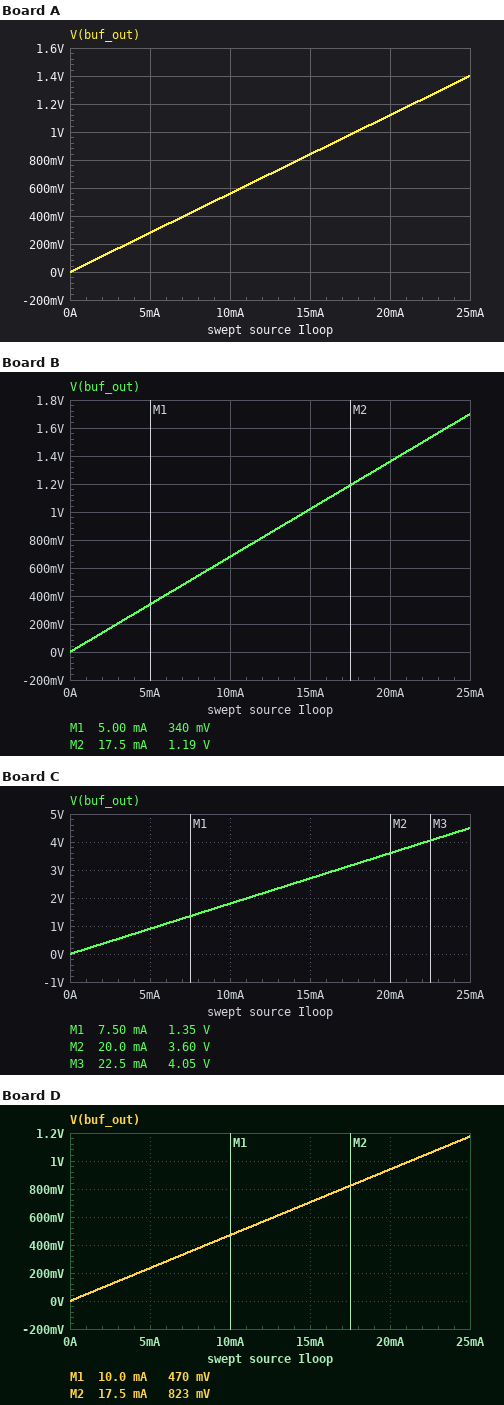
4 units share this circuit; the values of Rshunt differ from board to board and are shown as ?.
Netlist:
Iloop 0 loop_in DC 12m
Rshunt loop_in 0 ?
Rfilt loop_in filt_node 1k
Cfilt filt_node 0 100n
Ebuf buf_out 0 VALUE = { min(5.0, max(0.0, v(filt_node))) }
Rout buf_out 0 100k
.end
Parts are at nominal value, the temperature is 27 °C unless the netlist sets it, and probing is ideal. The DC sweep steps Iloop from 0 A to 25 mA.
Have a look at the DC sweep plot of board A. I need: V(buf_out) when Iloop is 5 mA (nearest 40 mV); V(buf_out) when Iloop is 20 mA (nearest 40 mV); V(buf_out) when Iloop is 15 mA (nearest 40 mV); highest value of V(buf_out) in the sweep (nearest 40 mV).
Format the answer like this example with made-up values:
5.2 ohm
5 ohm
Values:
280 mV
1.12 V
840 mV
1.40 V
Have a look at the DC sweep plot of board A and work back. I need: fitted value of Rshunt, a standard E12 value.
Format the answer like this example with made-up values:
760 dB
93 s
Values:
56 Ω
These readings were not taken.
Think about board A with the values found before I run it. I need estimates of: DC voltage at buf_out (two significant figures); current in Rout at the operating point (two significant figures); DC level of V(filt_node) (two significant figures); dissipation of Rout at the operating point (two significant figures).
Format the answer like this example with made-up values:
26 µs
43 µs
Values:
670 mV
6.7 µA
670 mV
4.5 µW
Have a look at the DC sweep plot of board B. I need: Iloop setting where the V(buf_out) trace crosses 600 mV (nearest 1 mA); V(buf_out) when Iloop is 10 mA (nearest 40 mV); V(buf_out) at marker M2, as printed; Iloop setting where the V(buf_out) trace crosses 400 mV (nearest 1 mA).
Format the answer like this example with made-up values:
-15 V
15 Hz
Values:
9 mA
680 mV
1.19 V
6 mA
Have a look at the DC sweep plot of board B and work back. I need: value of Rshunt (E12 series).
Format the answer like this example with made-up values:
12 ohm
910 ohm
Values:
68 Ω
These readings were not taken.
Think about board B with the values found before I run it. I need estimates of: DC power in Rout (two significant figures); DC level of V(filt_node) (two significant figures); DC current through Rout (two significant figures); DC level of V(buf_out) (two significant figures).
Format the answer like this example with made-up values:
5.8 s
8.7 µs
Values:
6.7 µW
820 mV
8.2 µA
820 mV
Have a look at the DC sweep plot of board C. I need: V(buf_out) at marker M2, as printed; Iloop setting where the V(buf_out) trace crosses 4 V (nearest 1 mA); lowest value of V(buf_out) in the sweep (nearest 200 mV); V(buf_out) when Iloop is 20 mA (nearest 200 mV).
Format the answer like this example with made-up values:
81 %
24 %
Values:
3.60 V
22 mA
0 V
3.6 V
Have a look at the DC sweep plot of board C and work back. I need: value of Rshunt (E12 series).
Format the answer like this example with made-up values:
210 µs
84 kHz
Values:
180 Ω
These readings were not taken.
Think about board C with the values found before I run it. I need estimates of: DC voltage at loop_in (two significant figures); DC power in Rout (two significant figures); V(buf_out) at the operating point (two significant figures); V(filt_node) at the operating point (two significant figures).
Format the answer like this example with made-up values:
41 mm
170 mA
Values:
2.2 V
47 µW
2.2 V
2.2 V
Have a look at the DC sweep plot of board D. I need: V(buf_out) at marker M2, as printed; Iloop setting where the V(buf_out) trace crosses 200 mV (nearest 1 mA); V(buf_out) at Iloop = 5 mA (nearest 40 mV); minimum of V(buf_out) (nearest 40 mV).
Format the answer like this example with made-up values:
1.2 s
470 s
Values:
823 mV
4 mA
240 mV
0 V
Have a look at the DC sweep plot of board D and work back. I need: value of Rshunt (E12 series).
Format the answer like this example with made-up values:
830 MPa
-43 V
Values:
47 Ω
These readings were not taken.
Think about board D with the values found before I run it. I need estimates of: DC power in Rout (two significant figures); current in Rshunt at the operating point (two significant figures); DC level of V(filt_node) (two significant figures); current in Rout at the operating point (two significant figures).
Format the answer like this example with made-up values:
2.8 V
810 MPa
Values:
3.2 µW
12 mA
560 mV
5.6 µA
